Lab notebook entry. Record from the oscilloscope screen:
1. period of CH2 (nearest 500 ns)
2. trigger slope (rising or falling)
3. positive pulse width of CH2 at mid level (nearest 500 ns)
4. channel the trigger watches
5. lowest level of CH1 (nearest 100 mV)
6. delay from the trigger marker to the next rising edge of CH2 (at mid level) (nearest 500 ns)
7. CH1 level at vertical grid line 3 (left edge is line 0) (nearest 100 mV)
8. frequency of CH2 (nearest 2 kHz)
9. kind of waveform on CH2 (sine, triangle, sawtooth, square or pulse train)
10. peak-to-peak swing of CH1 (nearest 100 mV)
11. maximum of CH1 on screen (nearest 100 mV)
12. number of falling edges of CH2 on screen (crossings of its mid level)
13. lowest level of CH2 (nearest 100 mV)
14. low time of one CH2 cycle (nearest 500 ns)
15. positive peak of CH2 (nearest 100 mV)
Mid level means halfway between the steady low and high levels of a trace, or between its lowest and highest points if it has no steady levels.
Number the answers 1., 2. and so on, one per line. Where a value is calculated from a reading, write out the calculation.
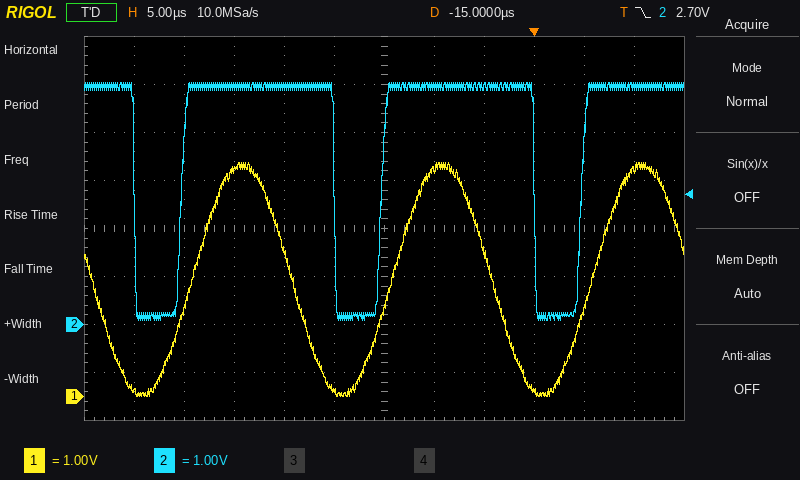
1. 20.0 µs
2. falling
3. 15.5 µs
4. CH2
5. 0.0 V
6. 4.5 µs
7. 4.7 V
8. 1 / 20.0 µs ≈ 50 kHz
9. pulse train
10. 4.9 V − (0.0 V) = 4.9 V
11. 4.9 V
12. 3
13. 100 mV
14. 4.5 µs
15. 5.0 V
